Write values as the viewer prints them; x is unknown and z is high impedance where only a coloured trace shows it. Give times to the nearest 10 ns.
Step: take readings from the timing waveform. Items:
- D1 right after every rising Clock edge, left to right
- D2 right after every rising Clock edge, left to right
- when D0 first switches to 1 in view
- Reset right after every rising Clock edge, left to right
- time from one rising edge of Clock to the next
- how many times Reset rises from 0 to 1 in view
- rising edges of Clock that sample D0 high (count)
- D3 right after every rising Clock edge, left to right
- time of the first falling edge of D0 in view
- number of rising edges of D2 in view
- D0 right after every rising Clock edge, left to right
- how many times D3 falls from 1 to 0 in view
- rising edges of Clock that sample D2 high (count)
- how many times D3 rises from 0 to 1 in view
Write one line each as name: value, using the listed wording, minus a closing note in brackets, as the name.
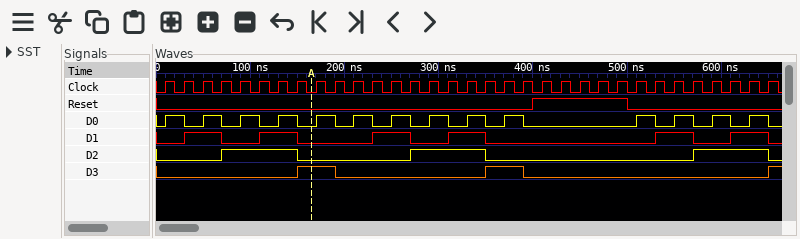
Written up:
D1 right after every rising Clock edge, left to right: 0 1 1 0 0 1 1 0 0 0 0 1 1 0 0 1 1 0 0 0 0 0 0 0 0 0 1 1 0 0 1 1 0
D2 right after every rising Clock edge, left to right: 0 0 0 1 1 1 1 0 0 0 0 0 0 1 1 1 1 0 0 0 0 0 0 0 0 0 0 0 1 1 1 1 0
when D0 first switches to 1 in view: 10 ns
Reset right after every rising Clock edge, left to right: 0 0 0 0 0 0 0 0 0 0 0 0 0 0 0 0 0 0 0 0 1 1 1 1 1 0 0 0 0 0 0 0 0
time from one rising edge of Clock to the next: 20 ns
how many times Reset rises from 0 to 1 in view: 1
rising edges of Clock that sample D0 high: 14
D3 right after every rising Clock edge, left to right: 0 0 0 0 0 0 0 1 1 0 0 0 0 0 0 0 0 1 1 0 0 0 0 0 0 0 0 0 0 0 0 0 1
time of the first falling edge of D0 in view: 30 ns
number of rising edges of D2 in view: 3
D0 right after every rising Clock edge, left to right: 1 0 1 0 1 0 1 0 1 0 1 0 1 0 1 0 1 0 1 0 0 0 0 0 0 1 0 1 0 1 0 1 0
how many times D3 falls from 1 to 0 in view: 2
rising edges of Clock that sample D2 high: 12
how many times D3 rises from 0 to 1 in view: 3
